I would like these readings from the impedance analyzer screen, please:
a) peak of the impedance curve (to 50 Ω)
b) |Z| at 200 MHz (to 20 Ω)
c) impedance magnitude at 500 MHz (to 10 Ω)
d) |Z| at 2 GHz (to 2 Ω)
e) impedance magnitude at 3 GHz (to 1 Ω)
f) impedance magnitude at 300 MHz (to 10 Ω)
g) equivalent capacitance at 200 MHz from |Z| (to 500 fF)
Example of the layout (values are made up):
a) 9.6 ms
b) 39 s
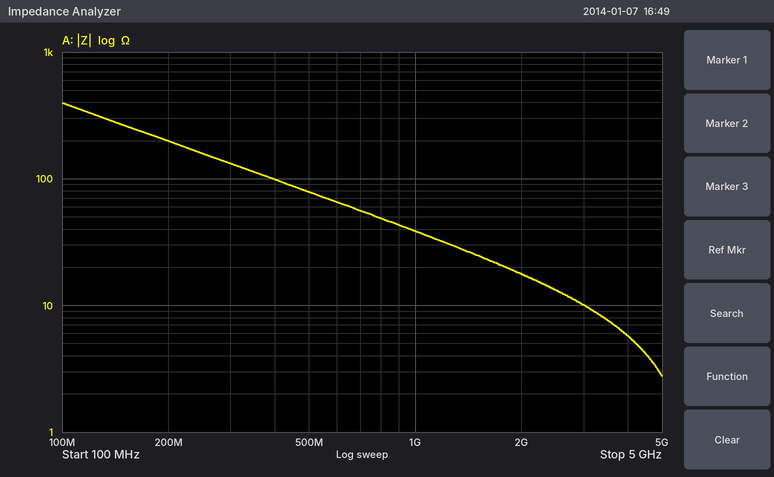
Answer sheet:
a) 400 Ω
b) 200 Ω
c) 80 Ω
d) 18 Ω
e) 10 Ω
f) 130 Ω
g) 4.0 pF
